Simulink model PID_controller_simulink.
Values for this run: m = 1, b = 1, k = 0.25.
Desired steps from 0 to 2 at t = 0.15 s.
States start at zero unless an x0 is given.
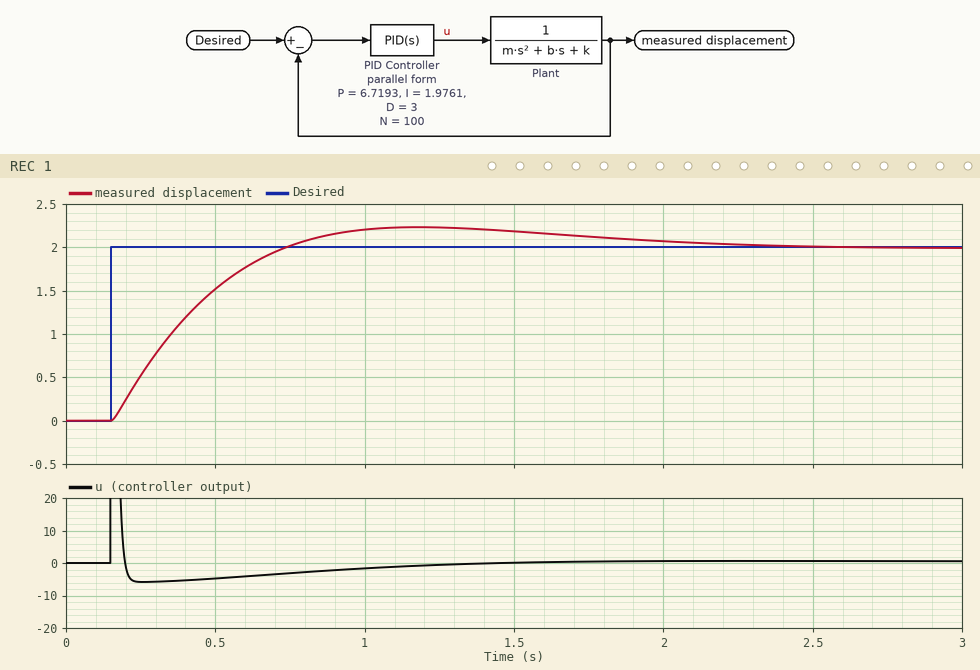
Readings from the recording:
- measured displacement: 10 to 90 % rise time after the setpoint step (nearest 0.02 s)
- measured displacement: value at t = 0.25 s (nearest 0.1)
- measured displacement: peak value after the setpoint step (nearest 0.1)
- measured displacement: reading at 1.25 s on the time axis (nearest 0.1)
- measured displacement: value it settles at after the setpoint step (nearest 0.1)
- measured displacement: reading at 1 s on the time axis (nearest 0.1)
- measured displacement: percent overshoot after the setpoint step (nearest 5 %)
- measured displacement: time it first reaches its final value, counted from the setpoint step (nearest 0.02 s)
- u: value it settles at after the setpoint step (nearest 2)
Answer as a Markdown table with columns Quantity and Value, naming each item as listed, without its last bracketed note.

| Quantity | Value |
|---|---|
| measured displacement: 10 to 90 % rise time after the setpoint step | 0.42 s |
| measured displacement: value at t = 0.25 s | 0.5 |
| measured displacement: peak value after the setpoint step | 2.2 |
| measured displacement: reading at 1.25 s on the time axis | 2.2 |
| measured displacement: value it settles at after the setpoint step | 2.0 |
| measured displacement: reading at 1 s on the time axis | 2.2 |
| measured displacement: percent overshoot after the setpoint step | 10 % |
| measured displacement: time it first reaches its final value, counted from the setpoint step | 0.58 s |
| u: value it settles at after the setpoint step | 0 |
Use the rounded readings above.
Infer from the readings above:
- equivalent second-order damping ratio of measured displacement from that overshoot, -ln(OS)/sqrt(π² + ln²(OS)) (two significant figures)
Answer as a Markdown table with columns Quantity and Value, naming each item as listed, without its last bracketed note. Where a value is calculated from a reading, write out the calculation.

| Quantity | Value |
|---|---|
| equivalent second-order damping ratio of measured displacement from that overshoot, -ln(OS)/sqrt(π² + ln²(OS)) | ln(0.1) = -2.303; 2.303 / sqrt(9.870 + 5.302) = 0.59 |
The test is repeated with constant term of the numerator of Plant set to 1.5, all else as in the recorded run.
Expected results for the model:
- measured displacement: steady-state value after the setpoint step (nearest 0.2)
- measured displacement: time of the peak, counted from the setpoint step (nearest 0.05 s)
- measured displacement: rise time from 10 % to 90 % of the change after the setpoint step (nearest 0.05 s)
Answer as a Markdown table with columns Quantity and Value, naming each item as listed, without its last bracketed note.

| Quantity | Value |
|---|---|
| measured displacement: steady-state value after the setpoint step | 2.0 |
| measured displacement: time of the peak, counted from the setpoint step | 0.80 s |
| measured displacement: rise time from 10 % to 90 % of the change after the setpoint step | 0.30 s |
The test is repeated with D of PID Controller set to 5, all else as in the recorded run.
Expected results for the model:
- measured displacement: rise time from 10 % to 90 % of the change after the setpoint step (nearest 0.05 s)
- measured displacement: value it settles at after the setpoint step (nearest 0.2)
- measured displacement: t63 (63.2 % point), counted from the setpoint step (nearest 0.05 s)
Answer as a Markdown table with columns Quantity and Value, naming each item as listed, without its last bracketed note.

| Quantity | Value |
|---|---|
| measured displacement: rise time from 10 % to 90 % of the change after the setpoint step | 0.35 s |
| measured displacement: value it settles at after the setpoint step | 2.0 |
| measured displacement: t63 (63.2 % point), counted from the setpoint step | 0.20 s |
